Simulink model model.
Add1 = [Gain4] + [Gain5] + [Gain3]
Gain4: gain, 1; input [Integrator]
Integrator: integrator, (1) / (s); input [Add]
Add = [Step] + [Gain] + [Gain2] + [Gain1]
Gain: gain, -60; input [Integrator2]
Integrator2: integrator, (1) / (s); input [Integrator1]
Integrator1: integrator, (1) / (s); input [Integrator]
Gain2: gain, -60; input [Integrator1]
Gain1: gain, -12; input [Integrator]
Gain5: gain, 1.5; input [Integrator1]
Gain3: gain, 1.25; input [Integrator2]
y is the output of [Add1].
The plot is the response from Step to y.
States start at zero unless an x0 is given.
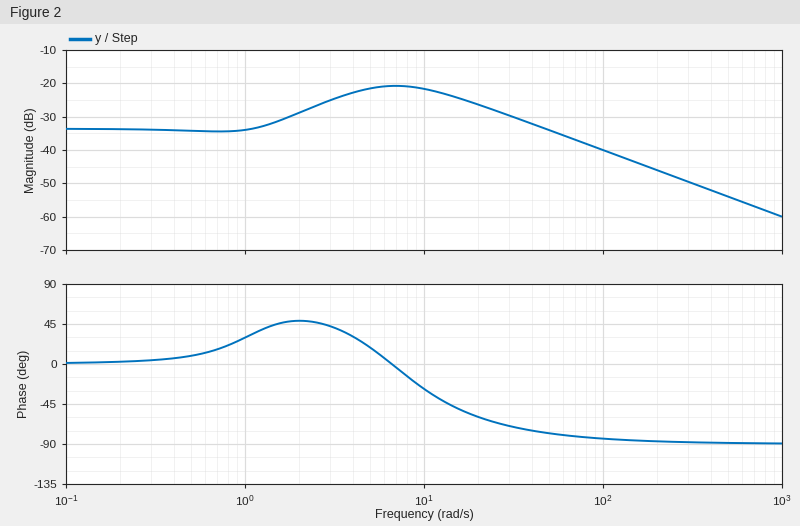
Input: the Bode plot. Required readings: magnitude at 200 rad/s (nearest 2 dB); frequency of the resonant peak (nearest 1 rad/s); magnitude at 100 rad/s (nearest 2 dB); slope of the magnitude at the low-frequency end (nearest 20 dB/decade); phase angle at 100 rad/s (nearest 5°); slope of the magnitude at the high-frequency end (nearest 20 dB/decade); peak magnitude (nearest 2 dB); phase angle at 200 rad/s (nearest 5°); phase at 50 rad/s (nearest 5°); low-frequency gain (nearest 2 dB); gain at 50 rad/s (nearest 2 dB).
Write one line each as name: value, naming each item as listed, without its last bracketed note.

magnitude at 200 rad/s: -46 dB
frequency of the resonant peak: 7 rad/s
magnitude at 100 rad/s: -40 dB
slope of the magnitude at the low-frequency end: 0 dB/decade
phase angle at 100 rad/s: -85°
slope of the magnitude at the high-frequency end: -20 dB/decade
peak magnitude: -20 dB
phase angle at 200 rad/s: -85°
phase at 50 rad/s: -80°
low-frequency gain: -34 dB
gain at 50 rad/s: -34 dB
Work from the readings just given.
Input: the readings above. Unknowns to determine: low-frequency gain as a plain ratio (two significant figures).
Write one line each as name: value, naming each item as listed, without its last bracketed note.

low-frequency gain as a plain ratio: 0.020
